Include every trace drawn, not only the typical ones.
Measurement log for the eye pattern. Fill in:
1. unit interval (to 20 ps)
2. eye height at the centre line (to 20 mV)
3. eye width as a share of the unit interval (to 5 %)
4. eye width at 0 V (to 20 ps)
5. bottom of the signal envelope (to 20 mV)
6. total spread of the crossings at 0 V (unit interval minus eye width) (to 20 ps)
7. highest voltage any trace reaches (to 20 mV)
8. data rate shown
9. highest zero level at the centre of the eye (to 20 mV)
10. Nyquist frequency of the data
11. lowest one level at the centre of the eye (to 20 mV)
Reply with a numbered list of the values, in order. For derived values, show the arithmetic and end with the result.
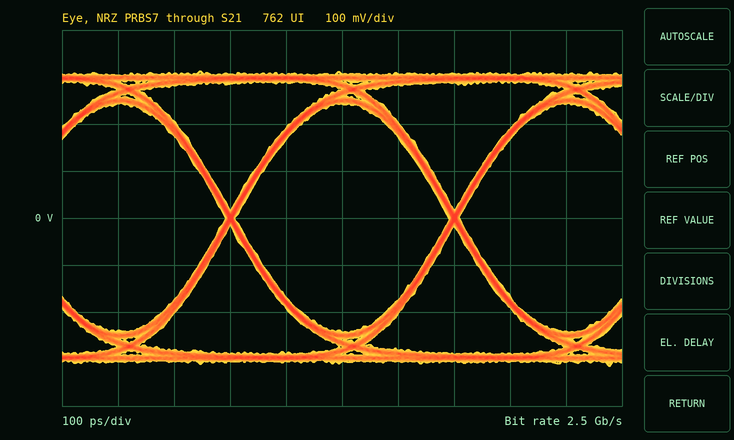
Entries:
1. 400 ps
2. 480 mV
3. 380 ps / 400 ps ≈ 95 %
4. 380 ps
5. -320 mV
6. 20 ps
7. 320 mV
8. 2.5 Gb/s
9. -240 mV
10. 1.25 GHz
11. 240 mV
